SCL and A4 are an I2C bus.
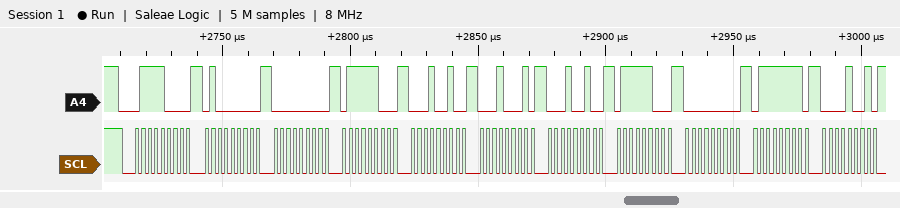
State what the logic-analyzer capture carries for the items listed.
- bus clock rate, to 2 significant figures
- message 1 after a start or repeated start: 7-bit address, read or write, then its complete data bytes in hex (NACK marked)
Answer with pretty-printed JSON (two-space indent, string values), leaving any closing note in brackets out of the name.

{
  "bus clock rate, to 2 significant figures": "400 kHz",
  "message 1 after a start or repeated start: 7-bit address, read or write, then its complete data bytes in hex": "0x3C write: 40 00 7C 12 11 12 7C 00 7F 09"
}
